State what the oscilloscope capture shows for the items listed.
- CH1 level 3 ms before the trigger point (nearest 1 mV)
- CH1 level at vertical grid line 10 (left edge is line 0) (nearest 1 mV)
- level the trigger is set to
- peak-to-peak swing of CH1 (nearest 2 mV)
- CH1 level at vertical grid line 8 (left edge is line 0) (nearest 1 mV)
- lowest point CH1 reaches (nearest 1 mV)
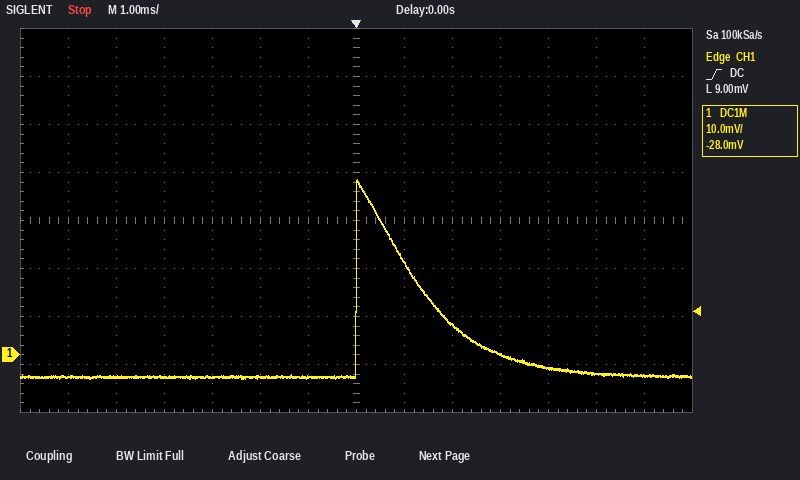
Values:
-5 mV
0 mV
9.00 mV
42 mV
19 mV
-5 mV
